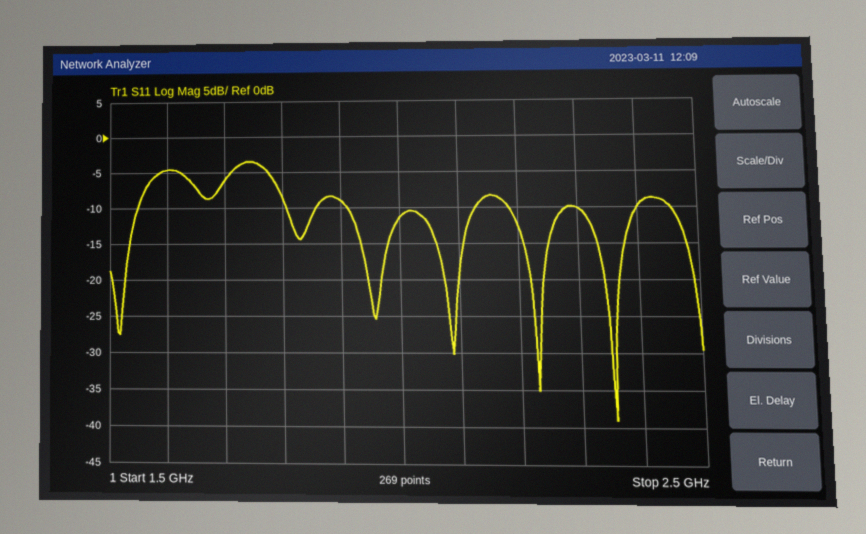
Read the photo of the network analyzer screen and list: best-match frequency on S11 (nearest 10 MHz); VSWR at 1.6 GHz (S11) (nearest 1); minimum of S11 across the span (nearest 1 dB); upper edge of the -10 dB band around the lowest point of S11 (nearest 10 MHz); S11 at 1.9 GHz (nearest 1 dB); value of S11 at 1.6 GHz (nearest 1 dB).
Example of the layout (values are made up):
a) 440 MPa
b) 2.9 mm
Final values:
a) 2.36 GHz
b) 4
c) -39 dB
d) 2.40 GHz
e) -9 dB
f) -5 dB
